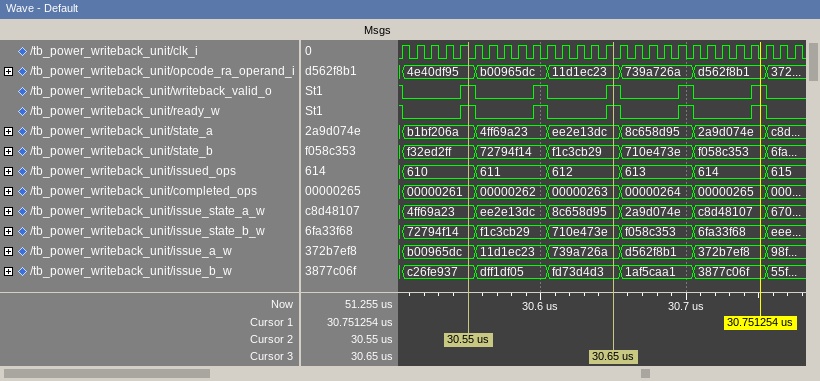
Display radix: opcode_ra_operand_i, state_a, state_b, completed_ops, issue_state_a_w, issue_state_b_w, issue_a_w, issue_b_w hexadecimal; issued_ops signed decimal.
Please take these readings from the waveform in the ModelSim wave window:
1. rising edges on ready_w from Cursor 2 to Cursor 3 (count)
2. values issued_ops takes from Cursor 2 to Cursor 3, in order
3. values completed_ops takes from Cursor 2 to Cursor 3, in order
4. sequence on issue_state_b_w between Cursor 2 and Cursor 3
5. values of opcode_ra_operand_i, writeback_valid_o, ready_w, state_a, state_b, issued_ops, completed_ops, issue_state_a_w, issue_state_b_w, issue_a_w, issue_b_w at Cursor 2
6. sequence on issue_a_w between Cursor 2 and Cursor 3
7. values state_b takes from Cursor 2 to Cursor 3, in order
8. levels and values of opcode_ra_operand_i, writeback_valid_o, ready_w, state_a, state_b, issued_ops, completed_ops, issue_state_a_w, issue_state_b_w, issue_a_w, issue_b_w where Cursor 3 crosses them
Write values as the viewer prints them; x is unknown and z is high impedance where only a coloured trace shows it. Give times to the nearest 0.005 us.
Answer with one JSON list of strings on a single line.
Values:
["2", "610, 611, 612", "00000261, 00000262, 00000263", "72794f14, f1c3cb29, 710e473e", "opcode_ra_operand_i=4e40df95, writeback_valid_o=1, ready_w=1, state_a=b1bf206a, state_b=f32ed2ff, issued_ops=610, completed_ops=00000261, issue_state_a_w=4ff69a23, issue_state_b_w=72794f14, issue_a_w=b00965dc, issue_b_w=c26fe937", "b00965dc, 11d1ec23, 739a726a", "f32ed2ff, 72794f14, f1c3cb29", "opcode_ra_operand_i=11d1ec23, writeback_valid_o=1, ready_w=1, state_a=ee2e13dc, state_b=f1c3cb29, issued_ops=612, completed_ops=00000263, issue_state_a_w=8c658d95, issue_state_b_w=710e473e, issue_a_w=739a726a, issue_b_w=fd73d4d3"]
